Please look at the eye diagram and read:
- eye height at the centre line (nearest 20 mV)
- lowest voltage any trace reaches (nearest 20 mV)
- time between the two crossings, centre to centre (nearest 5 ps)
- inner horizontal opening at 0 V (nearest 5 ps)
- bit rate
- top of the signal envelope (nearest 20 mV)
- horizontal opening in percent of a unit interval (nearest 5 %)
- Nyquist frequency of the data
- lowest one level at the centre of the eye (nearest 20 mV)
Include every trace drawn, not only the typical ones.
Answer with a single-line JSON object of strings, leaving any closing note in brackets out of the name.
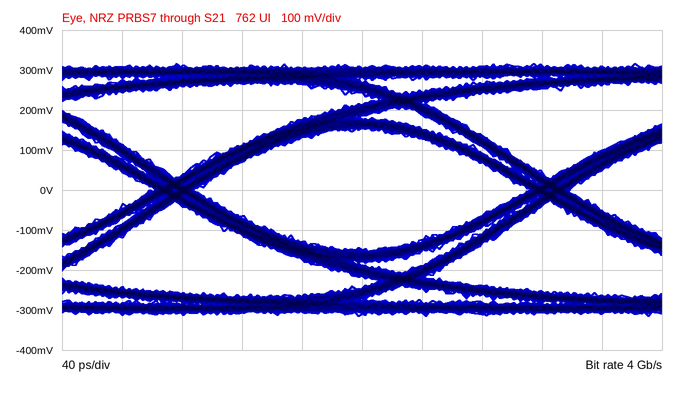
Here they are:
{"eye height at the centre line": "300 mV", "lowest voltage any trace reaches": "-320 mV", "time between the two crossings, centre to centre": "250 ps", "inner horizontal opening at 0 V": "225 ps", "bit rate": "4 Gb/s", "top of the signal envelope": "320 mV", "horizontal opening in percent of a unit interval": "90 %", "Nyquist frequency of the data": "2 GHz", "lowest one level at the centre of the eye": "160 mV"}
